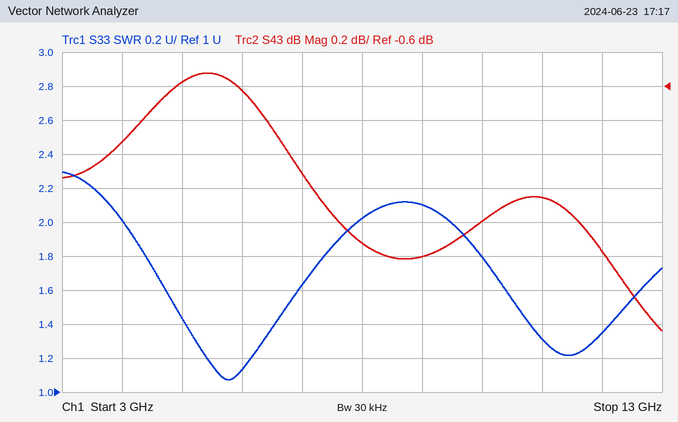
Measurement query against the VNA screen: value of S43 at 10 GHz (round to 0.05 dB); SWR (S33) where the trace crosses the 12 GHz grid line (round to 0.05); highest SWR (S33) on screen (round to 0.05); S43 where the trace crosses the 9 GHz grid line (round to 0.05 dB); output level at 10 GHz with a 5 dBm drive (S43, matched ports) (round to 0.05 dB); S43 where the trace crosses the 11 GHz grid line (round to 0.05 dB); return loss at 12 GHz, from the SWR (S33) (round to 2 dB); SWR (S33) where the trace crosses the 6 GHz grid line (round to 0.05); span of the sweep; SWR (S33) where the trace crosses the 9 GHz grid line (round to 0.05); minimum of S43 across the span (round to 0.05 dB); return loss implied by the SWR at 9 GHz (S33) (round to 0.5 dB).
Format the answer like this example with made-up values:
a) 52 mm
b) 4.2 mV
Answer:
a) -1.40 dB
b) 1.35
c) 2.30
d) -1.60 dB
e) 3.60 dBm
f) -1.25 dB
g) 16 dB
h) 1.15
i) 10 GHz
j) 2.10
k) -2.05 dB
l) 9.0 dB
